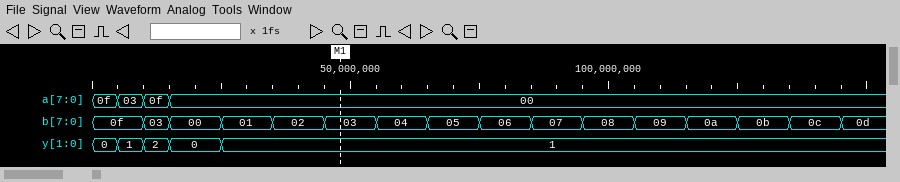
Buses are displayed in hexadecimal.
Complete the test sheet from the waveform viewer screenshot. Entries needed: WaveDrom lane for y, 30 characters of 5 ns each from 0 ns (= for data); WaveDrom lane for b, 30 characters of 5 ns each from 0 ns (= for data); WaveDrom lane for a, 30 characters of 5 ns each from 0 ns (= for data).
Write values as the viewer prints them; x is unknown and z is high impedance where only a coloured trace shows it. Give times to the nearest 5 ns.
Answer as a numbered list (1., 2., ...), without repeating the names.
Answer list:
1. {name: 'y', wave: '====.=........................', data: '0 1 2 0 1'}
2. {name: 'b', wave: '=.==.=.=.=.=.=.=.=.=.=.=.=.=.=', data: '0f 03 00 01 02 03 04 05 06 07 08 09 0a 0b 0c 0d'}
3. {name: 'a', wave: '====..........................', data: '0f 03 0f 00'}
